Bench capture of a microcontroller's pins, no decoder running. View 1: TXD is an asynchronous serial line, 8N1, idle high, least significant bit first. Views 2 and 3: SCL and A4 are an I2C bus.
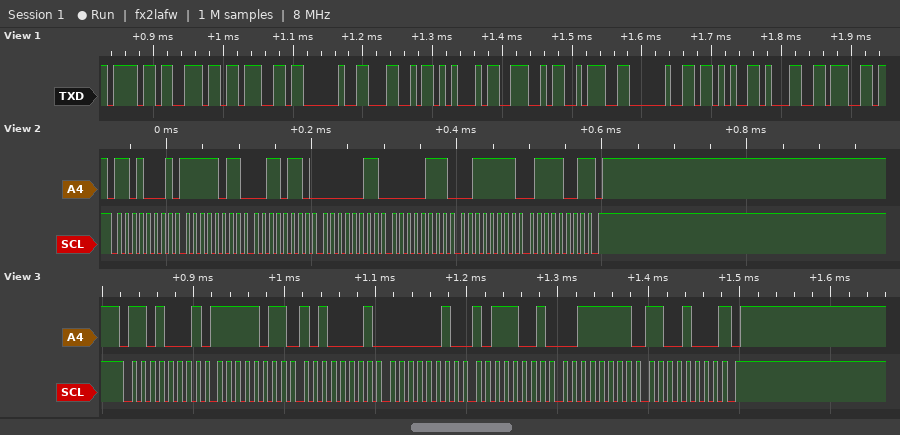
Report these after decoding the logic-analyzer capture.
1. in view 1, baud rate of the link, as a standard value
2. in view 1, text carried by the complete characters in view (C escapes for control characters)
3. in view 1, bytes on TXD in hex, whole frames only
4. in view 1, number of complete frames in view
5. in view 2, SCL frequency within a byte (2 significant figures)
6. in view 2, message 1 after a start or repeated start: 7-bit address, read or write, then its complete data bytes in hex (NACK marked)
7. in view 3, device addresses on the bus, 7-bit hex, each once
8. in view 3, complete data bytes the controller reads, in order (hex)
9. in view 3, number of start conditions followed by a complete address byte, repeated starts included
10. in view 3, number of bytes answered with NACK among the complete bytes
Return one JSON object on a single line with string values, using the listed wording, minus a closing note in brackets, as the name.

{"in view 1, baud rate of the link, as a standard value": "115200 baud", "in view 1, text carried by the complete characters in view": "\"ong LEN: +1g\"", "in view 1, bytes on TXD in hex, whole frames only": "0x6F 0x6E 0x67 0x20 0x4C 0x45 0x4E 0x3A 0x20 0x2B 0x31 0x67", "in view 1, number of complete frames in view": "12", "in view 2, SCL frequency within a byte": "100 kHz", "in view 2, message 1 after a start or repeated start: 7-bit address, read or write, then its complete data bytes in hex": "0x68 read: FB 36 03 07 3F 79 NACK", "in view 3, device addresses on the bus, 7-bit hex, each once": "0x68", "in view 3, complete data bytes the controller reads, in order": "FB A1 02 B9 3F C8", "in view 3, number of start conditions followed by a complete address byte, repeated starts included": "1", "in view 3, number of bytes answered with NACK among the complete bytes": "1"}
